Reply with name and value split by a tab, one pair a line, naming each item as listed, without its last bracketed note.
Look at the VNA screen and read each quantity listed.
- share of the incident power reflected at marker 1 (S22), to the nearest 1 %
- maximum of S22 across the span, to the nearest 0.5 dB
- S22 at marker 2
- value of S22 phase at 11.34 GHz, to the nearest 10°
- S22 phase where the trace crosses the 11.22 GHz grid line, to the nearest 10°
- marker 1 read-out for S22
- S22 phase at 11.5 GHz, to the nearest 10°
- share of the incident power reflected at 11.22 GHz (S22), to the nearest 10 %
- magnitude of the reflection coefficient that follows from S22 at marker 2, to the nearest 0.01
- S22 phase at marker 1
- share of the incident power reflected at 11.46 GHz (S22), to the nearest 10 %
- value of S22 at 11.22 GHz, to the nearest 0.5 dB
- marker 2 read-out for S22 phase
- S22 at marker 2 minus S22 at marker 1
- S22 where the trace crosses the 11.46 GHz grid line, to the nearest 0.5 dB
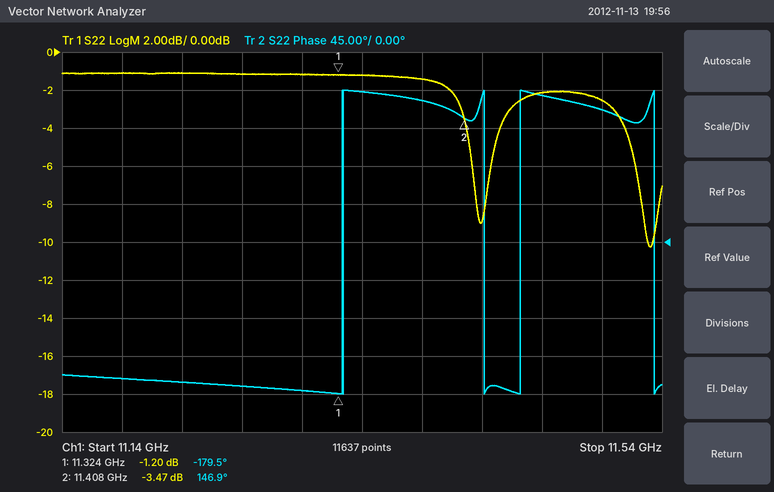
share of the incident power reflected at marker 1 (S22), to the nearest 1 %	76 %
maximum of S22 across the span, to the nearest 0.5 dB	-1.0 dB
S22 at marker 2	-3.47 dB
value of S22 phase at 11.34 GHz, to the nearest 10°	180°
S22 phase where the trace crosses the 11.22 GHz grid line, to the nearest 10°	-170°
marker 1 read-out for S22	-1.20 dB
S22 phase at 11.5 GHz, to the nearest 10°	160°
share of the incident power reflected at 11.22 GHz (S22), to the nearest 10 %	80 %
magnitude of the reflection coefficient that follows from S22 at marker 2, to the nearest 0.01	0.67
S22 phase at marker 1	-179.5°
share of the incident power reflected at 11.46 GHz (S22), to the nearest 10 %	60 %
value of S22 at 11.22 GHz, to the nearest 0.5 dB	-1.0 dB
marker 2 read-out for S22 phase	146.9°
S22 at marker 2 minus S22 at marker 1	-2.27 dB
S22 where the trace crosses the 11.46 GHz grid line, to the nearest 0.5 dB	-2.0 dB
